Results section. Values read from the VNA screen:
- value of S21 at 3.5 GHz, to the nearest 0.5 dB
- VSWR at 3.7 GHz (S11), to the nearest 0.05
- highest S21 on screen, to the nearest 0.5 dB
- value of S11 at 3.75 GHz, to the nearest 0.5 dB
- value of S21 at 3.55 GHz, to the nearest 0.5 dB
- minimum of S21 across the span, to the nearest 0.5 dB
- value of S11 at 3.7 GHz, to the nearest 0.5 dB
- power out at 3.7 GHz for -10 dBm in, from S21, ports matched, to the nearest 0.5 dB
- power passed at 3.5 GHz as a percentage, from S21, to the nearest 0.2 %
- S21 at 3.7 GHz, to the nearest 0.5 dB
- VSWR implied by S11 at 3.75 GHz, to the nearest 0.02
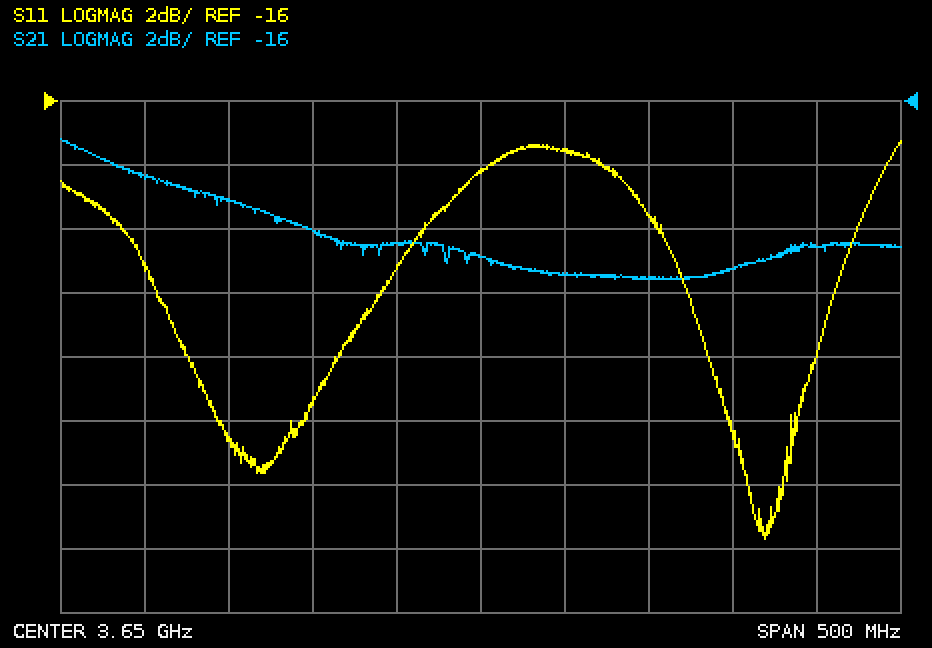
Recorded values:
-19.0 dB
1.30
-17.0 dB
-19.5 dB
-20.0 dB
-21.5 dB
-17.5 dB
-31.5 dBm
1.2 %
-21.5 dB
1.24
